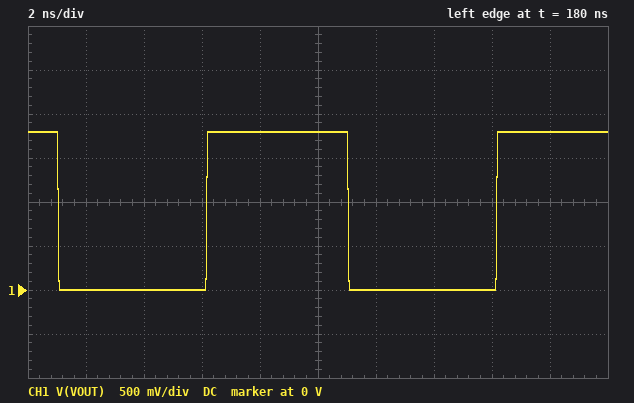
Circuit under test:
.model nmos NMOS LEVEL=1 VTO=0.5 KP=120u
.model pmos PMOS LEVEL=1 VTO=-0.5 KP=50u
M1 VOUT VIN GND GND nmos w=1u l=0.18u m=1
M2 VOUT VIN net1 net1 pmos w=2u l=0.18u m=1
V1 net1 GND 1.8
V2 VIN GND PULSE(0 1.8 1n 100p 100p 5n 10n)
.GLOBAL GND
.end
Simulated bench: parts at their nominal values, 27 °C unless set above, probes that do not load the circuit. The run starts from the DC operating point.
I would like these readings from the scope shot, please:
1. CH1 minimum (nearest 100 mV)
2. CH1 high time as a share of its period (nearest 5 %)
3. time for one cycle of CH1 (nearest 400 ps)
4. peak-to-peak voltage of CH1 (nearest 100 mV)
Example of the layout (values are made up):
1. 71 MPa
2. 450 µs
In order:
1. 0 V
2. 50 %
3. 10.0 ns
4. 1.8 V
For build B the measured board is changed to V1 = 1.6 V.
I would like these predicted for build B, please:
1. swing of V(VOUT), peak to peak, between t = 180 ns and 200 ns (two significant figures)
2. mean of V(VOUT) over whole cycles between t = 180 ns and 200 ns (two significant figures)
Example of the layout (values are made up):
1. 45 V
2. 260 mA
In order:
1. 1.6 V
2. 780 mV
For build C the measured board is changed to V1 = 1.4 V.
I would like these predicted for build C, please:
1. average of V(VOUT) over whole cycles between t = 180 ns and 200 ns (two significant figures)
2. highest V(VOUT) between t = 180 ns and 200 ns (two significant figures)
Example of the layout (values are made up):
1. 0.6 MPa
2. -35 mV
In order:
1. 680 mV
2. 1.4 V
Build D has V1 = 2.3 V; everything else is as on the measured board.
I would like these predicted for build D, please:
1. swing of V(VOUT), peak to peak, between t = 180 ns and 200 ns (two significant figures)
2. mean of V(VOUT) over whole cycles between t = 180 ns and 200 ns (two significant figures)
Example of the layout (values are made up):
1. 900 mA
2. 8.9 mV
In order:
1. 2.3 V
2. 1.1 V
